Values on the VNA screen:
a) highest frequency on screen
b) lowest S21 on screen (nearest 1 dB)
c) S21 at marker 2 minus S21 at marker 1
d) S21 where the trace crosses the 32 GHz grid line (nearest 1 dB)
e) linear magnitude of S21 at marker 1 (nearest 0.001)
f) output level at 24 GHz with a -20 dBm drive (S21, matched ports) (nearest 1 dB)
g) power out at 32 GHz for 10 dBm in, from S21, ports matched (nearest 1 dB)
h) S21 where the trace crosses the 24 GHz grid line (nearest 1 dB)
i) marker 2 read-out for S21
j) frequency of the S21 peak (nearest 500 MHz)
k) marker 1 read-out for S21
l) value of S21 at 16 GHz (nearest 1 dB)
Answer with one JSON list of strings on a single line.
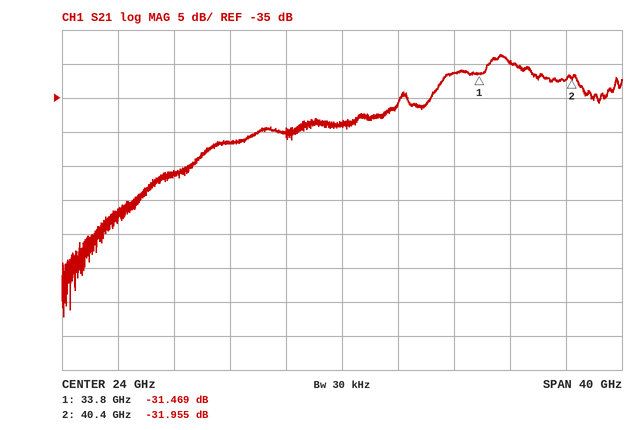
["44 GHz", "-67 dB", "-0.486 dB", "-31 dB", "0.027", "-59 dBm", "-21 dBm", "-39 dB", "-31.955 dB", "35.5 GHz", "-31.469 dB", "-42 dB"]
